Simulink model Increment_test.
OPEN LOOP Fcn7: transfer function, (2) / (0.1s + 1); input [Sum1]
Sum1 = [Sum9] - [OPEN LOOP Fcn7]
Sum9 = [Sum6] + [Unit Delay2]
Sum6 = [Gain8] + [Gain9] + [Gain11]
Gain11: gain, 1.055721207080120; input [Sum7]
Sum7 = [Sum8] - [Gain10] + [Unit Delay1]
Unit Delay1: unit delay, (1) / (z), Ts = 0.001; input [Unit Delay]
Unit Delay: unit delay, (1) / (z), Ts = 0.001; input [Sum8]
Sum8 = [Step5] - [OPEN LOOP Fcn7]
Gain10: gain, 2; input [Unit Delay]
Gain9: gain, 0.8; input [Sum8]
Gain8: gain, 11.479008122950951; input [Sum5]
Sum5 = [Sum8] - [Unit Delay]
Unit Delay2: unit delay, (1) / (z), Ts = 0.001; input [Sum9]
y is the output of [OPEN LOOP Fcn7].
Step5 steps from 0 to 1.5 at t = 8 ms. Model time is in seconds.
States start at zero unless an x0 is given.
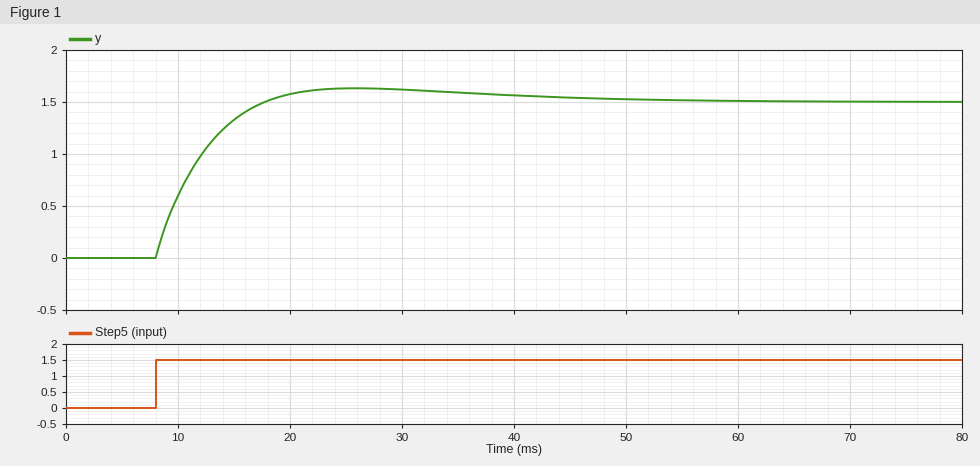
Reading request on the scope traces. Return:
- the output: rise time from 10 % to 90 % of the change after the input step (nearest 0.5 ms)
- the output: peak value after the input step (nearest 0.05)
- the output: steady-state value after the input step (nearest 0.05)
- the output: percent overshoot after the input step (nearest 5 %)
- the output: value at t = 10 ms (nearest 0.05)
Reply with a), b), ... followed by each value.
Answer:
a) 7.0 ms
b) 1.65
c) 1.50
d) 10 %
e) 0.60
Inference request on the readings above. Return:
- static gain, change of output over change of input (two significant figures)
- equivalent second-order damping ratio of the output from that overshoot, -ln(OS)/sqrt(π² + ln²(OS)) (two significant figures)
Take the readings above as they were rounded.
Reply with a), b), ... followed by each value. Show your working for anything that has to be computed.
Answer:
a) (1.5 - 0) / (1.5 - 0) = 1.0
b) ln(0.1) = -2.303; 2.303 / sqrt(9.870 + 5.302) = 0.59
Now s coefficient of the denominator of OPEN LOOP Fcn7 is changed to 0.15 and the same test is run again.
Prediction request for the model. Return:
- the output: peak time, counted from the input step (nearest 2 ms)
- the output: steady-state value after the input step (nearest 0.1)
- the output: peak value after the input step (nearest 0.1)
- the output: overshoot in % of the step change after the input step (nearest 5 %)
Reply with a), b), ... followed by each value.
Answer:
a) 22 ms
b) 1.5
c) 1.7
d) 15 %
